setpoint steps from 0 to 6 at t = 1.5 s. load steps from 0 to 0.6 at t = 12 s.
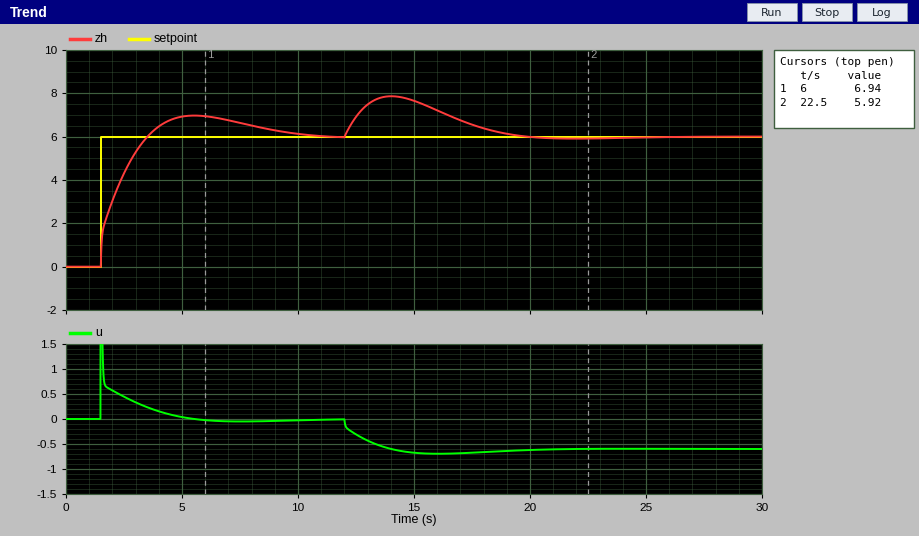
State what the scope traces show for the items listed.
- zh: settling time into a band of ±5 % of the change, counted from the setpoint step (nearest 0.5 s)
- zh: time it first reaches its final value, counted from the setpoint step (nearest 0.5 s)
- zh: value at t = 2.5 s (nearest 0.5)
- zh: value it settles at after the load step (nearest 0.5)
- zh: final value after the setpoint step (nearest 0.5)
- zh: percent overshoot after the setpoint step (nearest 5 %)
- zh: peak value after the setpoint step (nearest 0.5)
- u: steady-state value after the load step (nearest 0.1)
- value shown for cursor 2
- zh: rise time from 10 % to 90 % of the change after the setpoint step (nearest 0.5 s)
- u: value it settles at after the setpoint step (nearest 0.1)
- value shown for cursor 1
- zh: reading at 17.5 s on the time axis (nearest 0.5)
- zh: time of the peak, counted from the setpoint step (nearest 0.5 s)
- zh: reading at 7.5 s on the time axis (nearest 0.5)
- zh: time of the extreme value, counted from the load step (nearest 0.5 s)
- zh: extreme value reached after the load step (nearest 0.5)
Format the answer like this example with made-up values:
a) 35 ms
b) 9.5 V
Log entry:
a) 7.5 s
b) 2.0 s
c) 4.5
d) 6.0
e) 6.0
f) 15 %
g) 7.0
h) -0.6
i) 5.92
j) 1.5 s
k) 0.0
l) 6.94
m) 6.5
n) 4.0 s
o) 6.5
p) 2.0 s
q) 8.0
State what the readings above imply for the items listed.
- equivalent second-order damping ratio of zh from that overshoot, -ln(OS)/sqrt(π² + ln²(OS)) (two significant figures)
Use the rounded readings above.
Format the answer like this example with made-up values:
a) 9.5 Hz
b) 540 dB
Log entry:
a) 0.52
